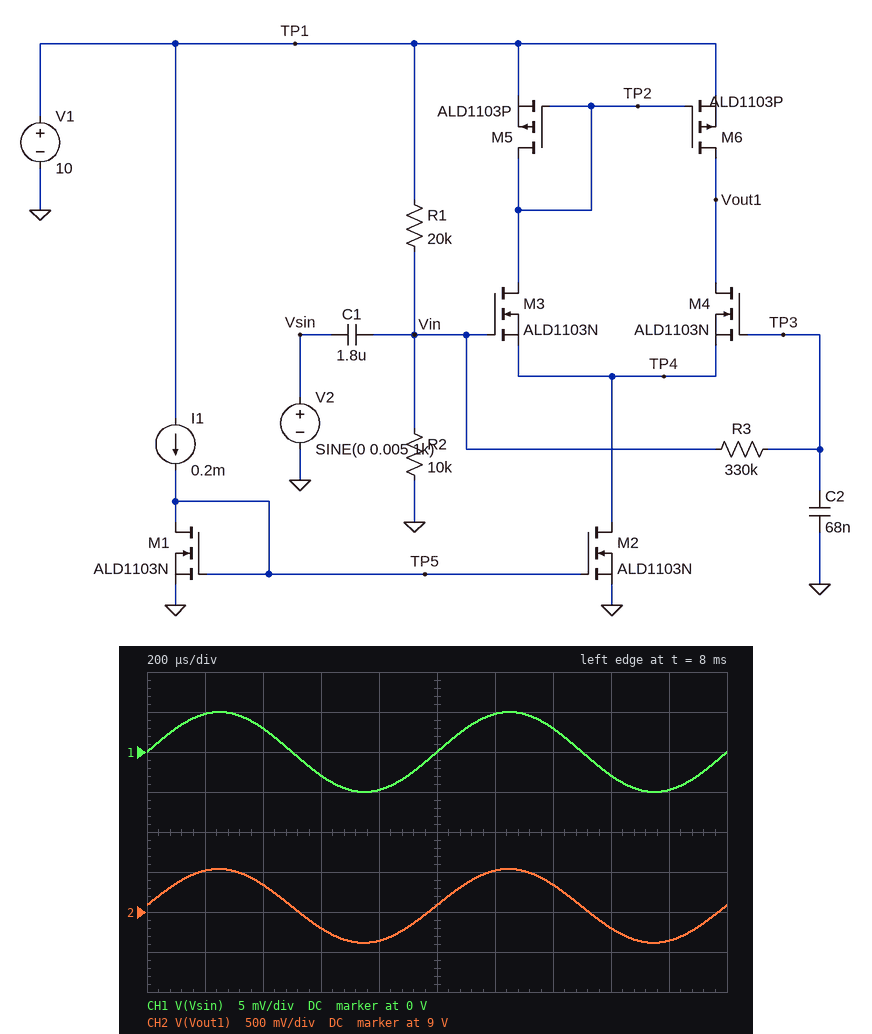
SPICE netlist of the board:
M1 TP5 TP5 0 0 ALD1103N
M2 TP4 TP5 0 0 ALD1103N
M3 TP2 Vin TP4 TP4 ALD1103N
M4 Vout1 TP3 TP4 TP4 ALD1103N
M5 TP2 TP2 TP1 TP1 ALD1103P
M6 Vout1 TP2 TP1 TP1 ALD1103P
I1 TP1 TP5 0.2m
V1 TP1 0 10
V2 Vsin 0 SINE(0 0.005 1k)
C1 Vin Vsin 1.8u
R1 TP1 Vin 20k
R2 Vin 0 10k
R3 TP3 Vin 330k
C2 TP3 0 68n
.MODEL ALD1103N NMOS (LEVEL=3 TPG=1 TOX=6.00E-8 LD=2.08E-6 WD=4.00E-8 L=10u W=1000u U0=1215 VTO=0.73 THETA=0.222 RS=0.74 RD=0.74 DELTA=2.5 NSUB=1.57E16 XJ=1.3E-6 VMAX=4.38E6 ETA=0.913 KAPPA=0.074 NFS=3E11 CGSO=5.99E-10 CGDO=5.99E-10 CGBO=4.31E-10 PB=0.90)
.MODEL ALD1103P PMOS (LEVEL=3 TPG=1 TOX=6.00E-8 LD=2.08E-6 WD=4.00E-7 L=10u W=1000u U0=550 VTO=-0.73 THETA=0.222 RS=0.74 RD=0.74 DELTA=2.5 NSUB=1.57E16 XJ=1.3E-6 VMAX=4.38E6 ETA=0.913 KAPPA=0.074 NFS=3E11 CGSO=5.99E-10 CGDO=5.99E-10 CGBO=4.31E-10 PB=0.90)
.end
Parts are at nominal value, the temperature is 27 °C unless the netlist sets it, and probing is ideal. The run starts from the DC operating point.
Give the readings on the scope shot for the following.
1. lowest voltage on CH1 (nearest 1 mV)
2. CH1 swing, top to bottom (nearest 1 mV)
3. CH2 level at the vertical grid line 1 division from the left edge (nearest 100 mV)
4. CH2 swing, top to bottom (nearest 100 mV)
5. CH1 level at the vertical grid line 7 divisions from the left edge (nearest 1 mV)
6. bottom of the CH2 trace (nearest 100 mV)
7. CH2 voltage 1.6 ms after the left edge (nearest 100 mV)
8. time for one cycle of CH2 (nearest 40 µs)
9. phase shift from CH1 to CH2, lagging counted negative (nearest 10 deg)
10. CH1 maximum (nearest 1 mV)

-5 mV
10 mV
9.5 V
900 mV
3 mV
8.6 V
8.8 V
1.00 ms
0 deg
5 mV
